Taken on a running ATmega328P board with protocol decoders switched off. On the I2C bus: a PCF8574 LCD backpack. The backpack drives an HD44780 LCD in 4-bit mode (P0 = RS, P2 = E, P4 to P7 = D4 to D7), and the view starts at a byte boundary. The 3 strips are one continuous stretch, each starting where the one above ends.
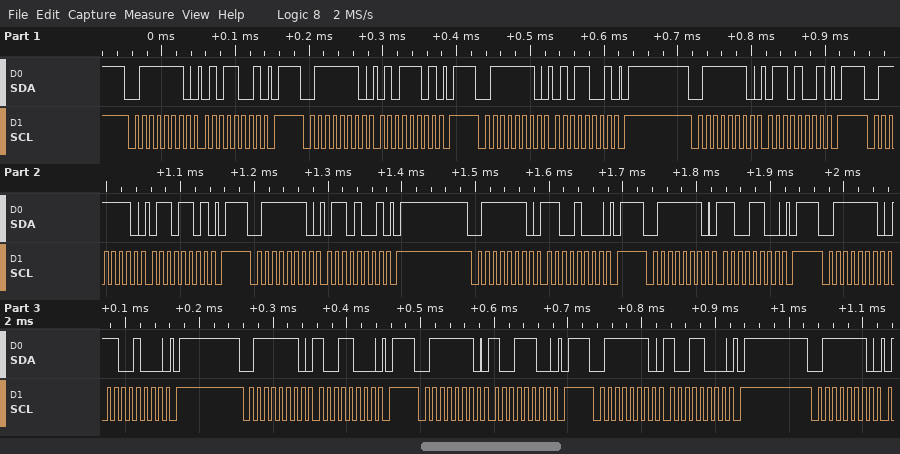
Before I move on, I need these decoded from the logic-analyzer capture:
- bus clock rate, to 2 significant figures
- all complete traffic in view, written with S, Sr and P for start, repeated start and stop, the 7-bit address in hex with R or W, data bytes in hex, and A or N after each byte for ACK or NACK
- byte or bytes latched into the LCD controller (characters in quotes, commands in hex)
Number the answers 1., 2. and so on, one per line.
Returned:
1. 100 kHz
2. S 3FW A 59 A P S 3FW A 5D A P S 3FW A 59 A P S 3FW A 69 A P S 3FW A 6D A P S 3FW A 69 A P S 3FW A C8 A P S 3FW A CC A P S 3FW A C8 A P S 3FW A 98 A P S 3FW A 9C A P S 3FW A 98 A P S 3FW A
3. 'V' 0xC9
